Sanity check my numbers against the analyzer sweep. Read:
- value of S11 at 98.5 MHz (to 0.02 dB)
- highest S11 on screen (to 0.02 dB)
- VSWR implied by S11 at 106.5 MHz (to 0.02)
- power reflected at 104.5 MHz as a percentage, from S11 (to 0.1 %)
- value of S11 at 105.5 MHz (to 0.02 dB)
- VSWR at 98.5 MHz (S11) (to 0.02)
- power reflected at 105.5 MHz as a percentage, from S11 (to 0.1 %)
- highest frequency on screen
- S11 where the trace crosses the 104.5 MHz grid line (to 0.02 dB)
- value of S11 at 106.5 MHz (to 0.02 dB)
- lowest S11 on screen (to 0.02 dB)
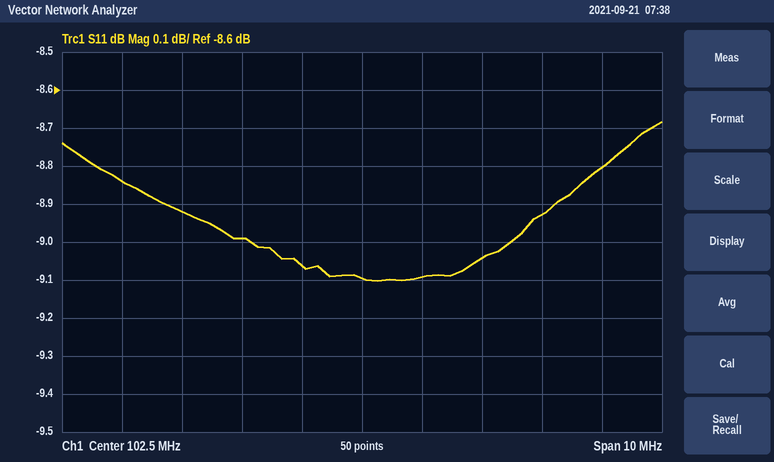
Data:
-8.84 dB
-8.68 dB
2.14
12.5 %
-8.92 dB
2.14
12.8 %
107.5 MHz
-9.04 dB
-8.80 dB
-9.10 dB
